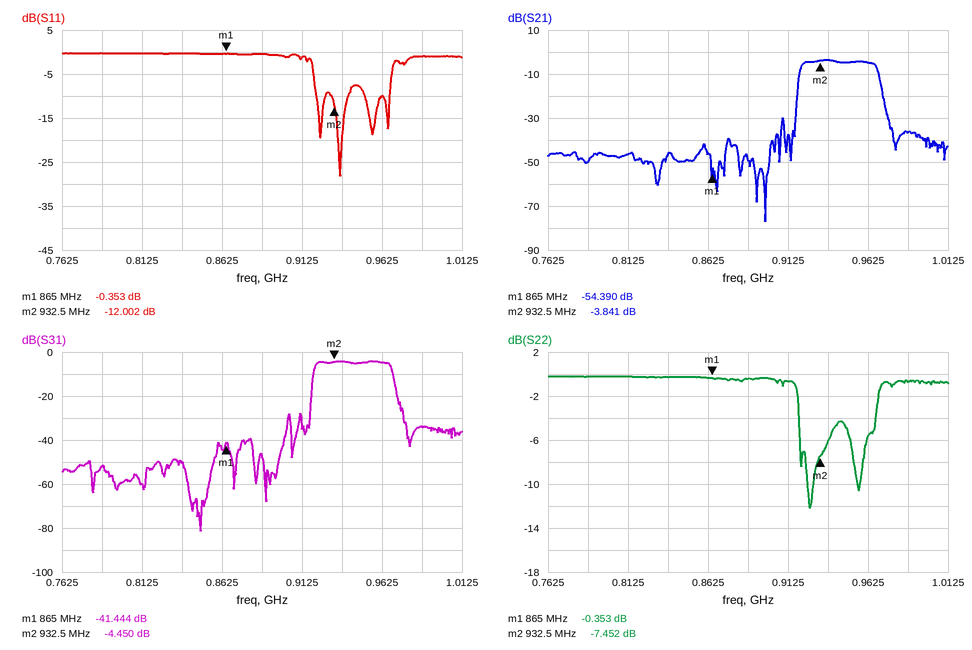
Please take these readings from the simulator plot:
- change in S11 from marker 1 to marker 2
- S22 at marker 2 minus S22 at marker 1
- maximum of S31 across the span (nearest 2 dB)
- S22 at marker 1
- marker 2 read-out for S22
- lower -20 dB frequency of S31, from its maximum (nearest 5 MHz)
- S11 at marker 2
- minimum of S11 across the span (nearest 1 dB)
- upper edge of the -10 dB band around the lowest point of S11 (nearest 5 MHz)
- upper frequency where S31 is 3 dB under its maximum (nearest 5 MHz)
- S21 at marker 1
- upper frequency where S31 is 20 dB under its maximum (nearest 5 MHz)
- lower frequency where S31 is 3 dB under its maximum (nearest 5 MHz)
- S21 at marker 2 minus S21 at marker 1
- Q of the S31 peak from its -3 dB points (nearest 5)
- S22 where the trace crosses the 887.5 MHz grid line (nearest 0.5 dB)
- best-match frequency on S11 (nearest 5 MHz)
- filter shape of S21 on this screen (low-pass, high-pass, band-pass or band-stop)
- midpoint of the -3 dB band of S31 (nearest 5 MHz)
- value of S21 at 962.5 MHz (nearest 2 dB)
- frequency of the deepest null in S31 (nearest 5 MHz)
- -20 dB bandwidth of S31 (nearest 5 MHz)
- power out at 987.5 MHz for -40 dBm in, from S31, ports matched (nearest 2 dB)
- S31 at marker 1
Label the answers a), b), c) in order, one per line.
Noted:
a) -11.649 dB
b) -7.099 dB
c) -4 dB
d) -0.353 dB
e) -7.452 dB
f) 920 MHz
g) -12.002 dB
h) -28 dB
i) 940 MHz
j) 970 MHz
k) -54.390 dB
l) 975 MHz
m) 920 MHz
n) 50.549 dB
o) 20
p) -0.5 dB
q) 935 MHz
r) band-pass
s) 945 MHz
t) -4 dB
u) 850 MHz
v) 55 MHz
w) -74 dBm
x) -41.444 dB
